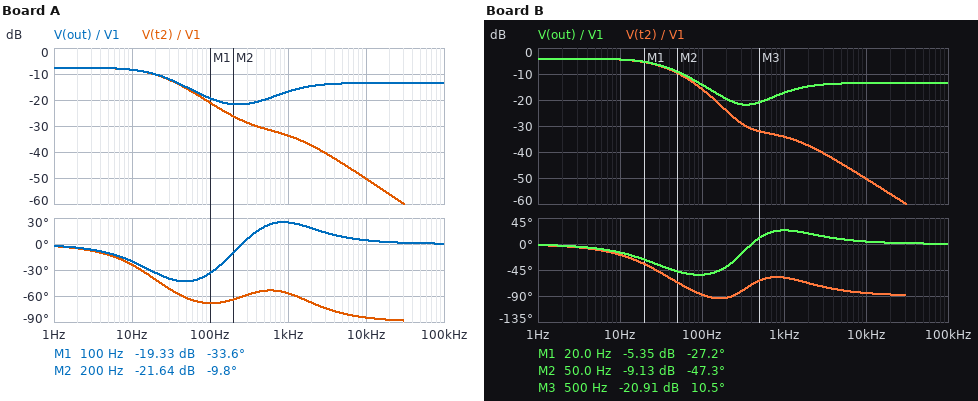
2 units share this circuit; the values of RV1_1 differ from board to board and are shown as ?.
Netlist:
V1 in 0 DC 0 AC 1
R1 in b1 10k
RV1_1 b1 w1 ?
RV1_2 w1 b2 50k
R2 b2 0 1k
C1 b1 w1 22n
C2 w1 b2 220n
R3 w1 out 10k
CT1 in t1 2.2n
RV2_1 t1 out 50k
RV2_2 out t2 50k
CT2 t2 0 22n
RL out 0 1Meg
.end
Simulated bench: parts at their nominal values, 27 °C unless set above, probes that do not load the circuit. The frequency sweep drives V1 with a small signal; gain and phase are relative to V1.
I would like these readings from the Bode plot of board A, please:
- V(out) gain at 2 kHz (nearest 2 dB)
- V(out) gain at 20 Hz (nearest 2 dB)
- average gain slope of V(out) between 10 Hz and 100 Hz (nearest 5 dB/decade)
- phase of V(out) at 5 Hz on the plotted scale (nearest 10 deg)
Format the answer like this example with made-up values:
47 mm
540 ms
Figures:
-14 dB
-10 dB
-10 dB/decade
-10 deg
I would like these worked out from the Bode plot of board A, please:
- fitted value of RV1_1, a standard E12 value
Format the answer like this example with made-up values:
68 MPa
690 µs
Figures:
56 kΩ
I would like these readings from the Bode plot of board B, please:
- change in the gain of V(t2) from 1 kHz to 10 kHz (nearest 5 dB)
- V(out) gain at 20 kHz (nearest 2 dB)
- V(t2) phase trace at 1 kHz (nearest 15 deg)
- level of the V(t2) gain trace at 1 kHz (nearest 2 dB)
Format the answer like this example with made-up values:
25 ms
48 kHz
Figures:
-15 dB
-14 dB
-60 deg
-34 dB
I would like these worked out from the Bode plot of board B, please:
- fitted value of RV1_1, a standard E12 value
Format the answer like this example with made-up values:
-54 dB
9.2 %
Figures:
18 kΩ
